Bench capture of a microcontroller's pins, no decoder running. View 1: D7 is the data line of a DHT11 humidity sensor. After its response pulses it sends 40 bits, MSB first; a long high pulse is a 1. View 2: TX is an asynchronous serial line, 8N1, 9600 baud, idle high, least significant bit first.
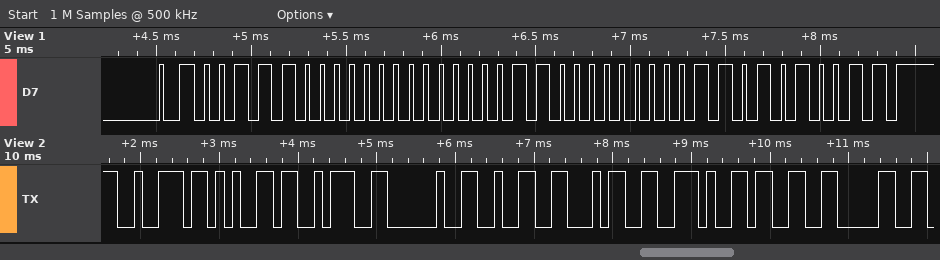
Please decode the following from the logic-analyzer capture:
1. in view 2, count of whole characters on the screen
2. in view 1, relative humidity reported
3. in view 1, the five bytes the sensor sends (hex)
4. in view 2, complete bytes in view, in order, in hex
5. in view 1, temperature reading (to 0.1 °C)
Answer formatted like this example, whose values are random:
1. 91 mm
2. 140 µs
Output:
1. 9
2. 56 %
3. 38 00 18 03 53
4. 0x72 0x65 0x3A 0x20 0x32 0x34 0x2E 0x33 0x30
5. 24.3 °C
